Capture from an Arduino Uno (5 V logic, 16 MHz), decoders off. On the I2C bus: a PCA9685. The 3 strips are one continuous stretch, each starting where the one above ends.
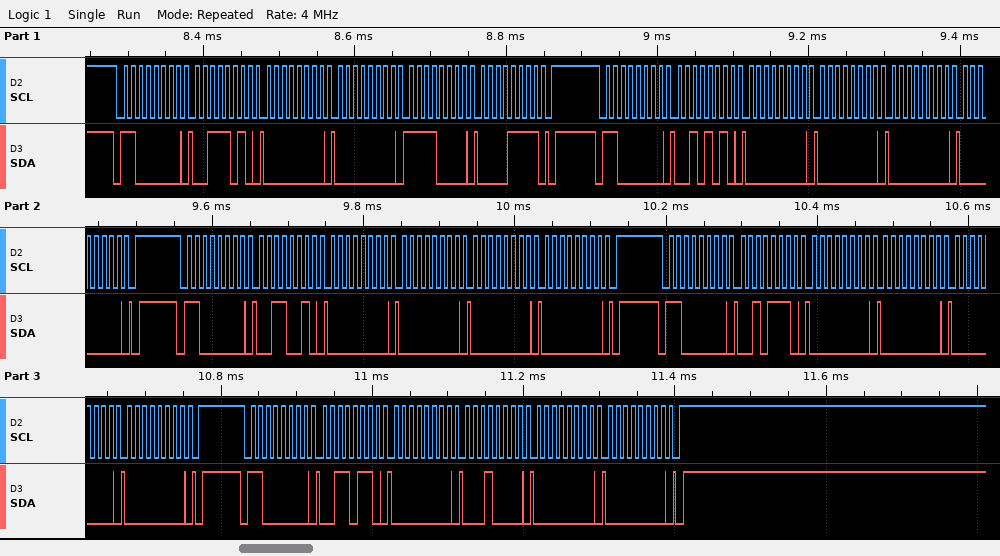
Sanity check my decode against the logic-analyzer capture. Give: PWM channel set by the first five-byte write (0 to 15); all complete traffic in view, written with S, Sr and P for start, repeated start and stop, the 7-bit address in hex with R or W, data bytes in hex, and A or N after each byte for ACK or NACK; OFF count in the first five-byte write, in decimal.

13
S 60W A 3A A 00 A 00 A F0 A 0F A P S 60W A 2A A 00 A 00 A 00 A 00 A P S 60W A 32 A 00 A 00 A 00 A 00 A P S 60W A 2E A 00 A 00 A 00 A 00 A P S 60W A 36 A 00 A 10 A 00 A 00 A P
4080
